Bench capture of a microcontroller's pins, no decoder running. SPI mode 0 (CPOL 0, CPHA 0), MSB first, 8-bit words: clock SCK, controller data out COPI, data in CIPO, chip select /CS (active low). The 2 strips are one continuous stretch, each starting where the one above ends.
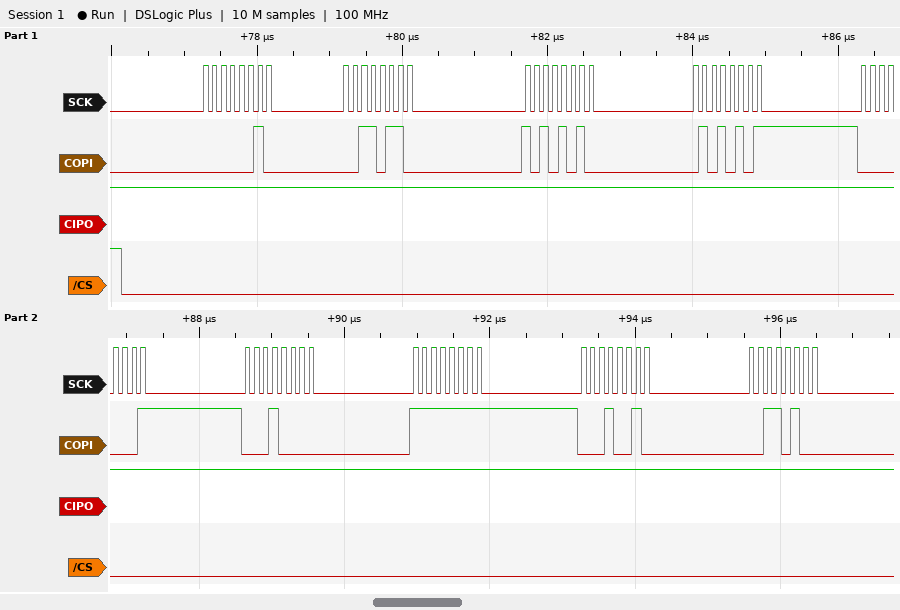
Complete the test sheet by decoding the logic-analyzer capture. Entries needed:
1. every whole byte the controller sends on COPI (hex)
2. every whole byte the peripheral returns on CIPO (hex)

02 36 AA 55 01 10 FF 12 34
FF FF FF FF FF FF FF FF FF
